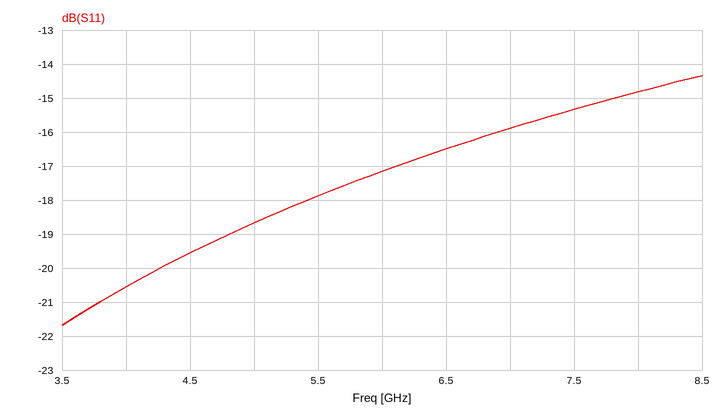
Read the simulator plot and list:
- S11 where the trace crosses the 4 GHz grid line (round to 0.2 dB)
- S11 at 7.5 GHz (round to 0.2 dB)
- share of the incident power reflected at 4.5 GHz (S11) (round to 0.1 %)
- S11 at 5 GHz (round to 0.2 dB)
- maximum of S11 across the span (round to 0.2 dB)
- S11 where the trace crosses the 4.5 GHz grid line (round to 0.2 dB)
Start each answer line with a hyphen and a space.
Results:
- -20.6 dB
- -15.4 dB
- 1.1 %
- -18.6 dB
- -14.4 dB
- -19.6 dB
